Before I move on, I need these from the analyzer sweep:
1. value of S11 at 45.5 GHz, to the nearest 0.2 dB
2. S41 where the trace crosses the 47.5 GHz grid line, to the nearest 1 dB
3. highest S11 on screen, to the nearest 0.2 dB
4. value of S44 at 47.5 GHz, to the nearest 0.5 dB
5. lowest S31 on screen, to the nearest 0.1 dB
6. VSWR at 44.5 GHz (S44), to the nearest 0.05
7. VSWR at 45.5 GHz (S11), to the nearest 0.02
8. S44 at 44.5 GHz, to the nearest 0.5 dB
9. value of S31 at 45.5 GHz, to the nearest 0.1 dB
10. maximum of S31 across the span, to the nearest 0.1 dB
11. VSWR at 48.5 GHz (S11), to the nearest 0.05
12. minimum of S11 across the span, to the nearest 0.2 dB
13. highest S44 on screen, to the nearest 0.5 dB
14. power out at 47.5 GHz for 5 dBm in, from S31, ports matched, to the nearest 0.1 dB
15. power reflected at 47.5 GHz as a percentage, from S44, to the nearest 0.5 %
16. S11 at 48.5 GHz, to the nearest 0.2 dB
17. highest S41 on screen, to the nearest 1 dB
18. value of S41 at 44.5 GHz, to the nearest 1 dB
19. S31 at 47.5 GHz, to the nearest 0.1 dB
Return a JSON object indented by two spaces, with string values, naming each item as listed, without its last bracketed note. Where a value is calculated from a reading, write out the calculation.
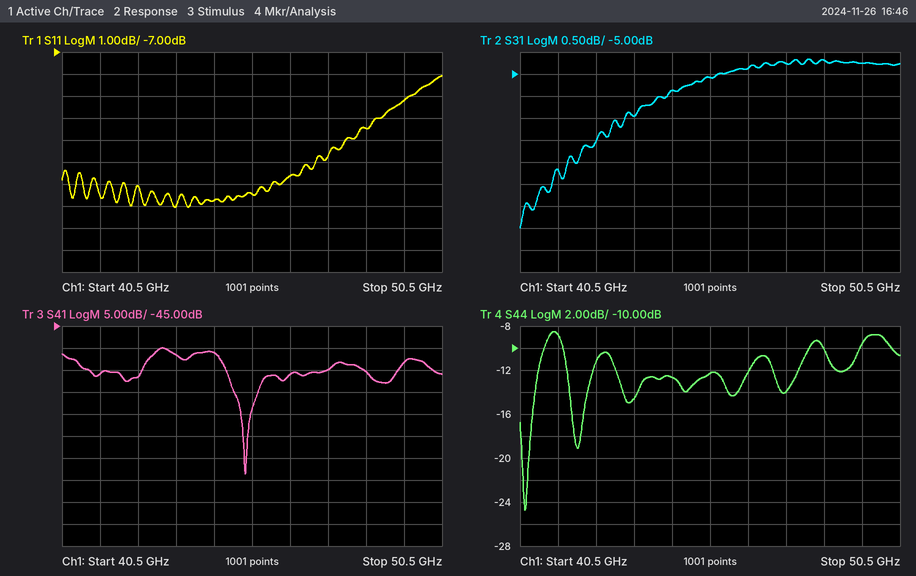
{
  "value of S11 at 45.5 GHz, to the nearest 0.2 dB": "-13.4 dB",
  "S41 where the trace crosses the 47.5 GHz grid line, to the nearest 1 dB": "-55 dB",
  "highest S11 on screen, to the nearest 0.2 dB": "-8.0 dB",
  "value of S44 at 47.5 GHz, to the nearest 0.5 dB": "-14.0 dB",
  "lowest S31 on screen, to the nearest 0.1 dB": "-8.5 dB",
  "VSWR at 44.5 GHz (S44), to the nearest 0.05": "|Γ| = 10^(-12.5/20) = 0.2371; VSWR = (1 + 0.2371)/(1 − 0.2371) ≈ 1.62, so 1.60 to the nearest 0.05",
  "VSWR at 45.5 GHz (S11), to the nearest 0.02": "|Γ| = 10^(-13.4/20) = 0.2138; VSWR = (1 + 0.2138)/(1 − 0.2138) ≈ 1.54",
  "S44 at 44.5 GHz, to the nearest 0.5 dB": "-12.5 dB",
  "value of S31 at 45.5 GHz, to the nearest 0.1 dB": "-5.1 dB",
  "maximum of S31 across the span, to the nearest 0.1 dB": "-4.7 dB",
  "VSWR at 48.5 GHz (S11), to the nearest 0.05": "|Γ| = 10^(-10.4/20) = 0.3020; VSWR = (1 + 0.3020)/(1 − 0.3020) ≈ 1.87, so 1.85 to the nearest 0.05",
  "minimum of S11 across the span, to the nearest 0.2 dB": "-14.0 dB",
  "highest S44 on screen, to the nearest 0.5 dB": "-8.5 dB",
  "power out at 47.5 GHz for 5 dBm in, from S31, ports matched, to the nearest 0.1 dB": "5 dBm + (-4.8 dB) = 0.2 dBm",
  "power reflected at 47.5 GHz as a percentage, from S44, to the nearest 0.5 %": "10^(-14/10) ≈ 4.0 %",
  "S11 at 48.5 GHz, to the nearest 0.2 dB": "-10.4 dB",
  "highest S41 on screen, to the nearest 1 dB": "-50 dB",
  "value of S41 at 44.5 GHz, to the nearest 1 dB": "-51 dB",
  "S31 at 47.5 GHz, to the nearest 0.1 dB": "-4.8 dB"
}
